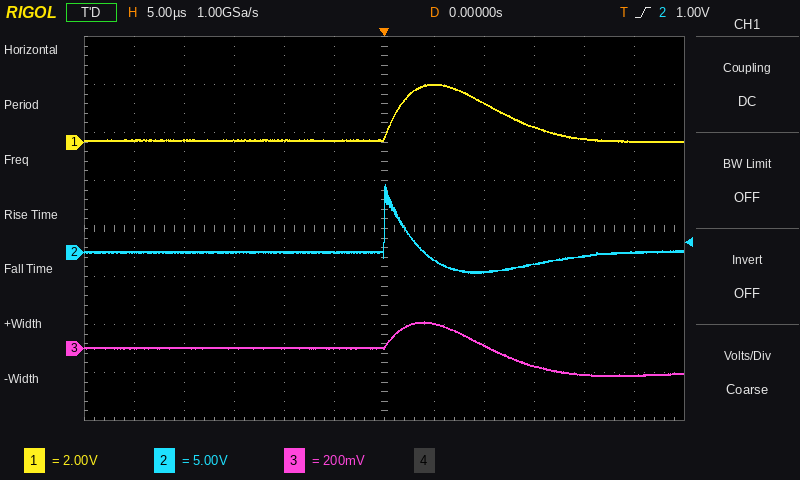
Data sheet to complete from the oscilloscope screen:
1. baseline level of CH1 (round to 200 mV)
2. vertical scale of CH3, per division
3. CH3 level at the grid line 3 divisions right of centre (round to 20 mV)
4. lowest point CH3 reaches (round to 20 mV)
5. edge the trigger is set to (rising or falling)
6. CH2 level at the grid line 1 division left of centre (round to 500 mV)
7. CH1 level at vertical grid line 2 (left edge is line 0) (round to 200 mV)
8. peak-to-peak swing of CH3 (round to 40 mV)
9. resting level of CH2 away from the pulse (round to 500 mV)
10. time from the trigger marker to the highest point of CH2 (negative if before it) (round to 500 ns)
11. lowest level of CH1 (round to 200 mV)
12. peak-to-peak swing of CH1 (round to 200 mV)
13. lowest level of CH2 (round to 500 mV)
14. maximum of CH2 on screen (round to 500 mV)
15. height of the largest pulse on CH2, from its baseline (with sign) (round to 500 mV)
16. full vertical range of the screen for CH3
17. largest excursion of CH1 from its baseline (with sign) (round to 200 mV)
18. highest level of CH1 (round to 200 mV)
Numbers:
0.0 V
200 mV
-80 mV
-120 mV
rising
0.0 V
0.0 V
240 mV
0.0 V
0.0 µs
0.0 V
2.4 V
-2.0 V
7.0 V
+7.0 V
1.6 V
+2.4 V
2.4 V
